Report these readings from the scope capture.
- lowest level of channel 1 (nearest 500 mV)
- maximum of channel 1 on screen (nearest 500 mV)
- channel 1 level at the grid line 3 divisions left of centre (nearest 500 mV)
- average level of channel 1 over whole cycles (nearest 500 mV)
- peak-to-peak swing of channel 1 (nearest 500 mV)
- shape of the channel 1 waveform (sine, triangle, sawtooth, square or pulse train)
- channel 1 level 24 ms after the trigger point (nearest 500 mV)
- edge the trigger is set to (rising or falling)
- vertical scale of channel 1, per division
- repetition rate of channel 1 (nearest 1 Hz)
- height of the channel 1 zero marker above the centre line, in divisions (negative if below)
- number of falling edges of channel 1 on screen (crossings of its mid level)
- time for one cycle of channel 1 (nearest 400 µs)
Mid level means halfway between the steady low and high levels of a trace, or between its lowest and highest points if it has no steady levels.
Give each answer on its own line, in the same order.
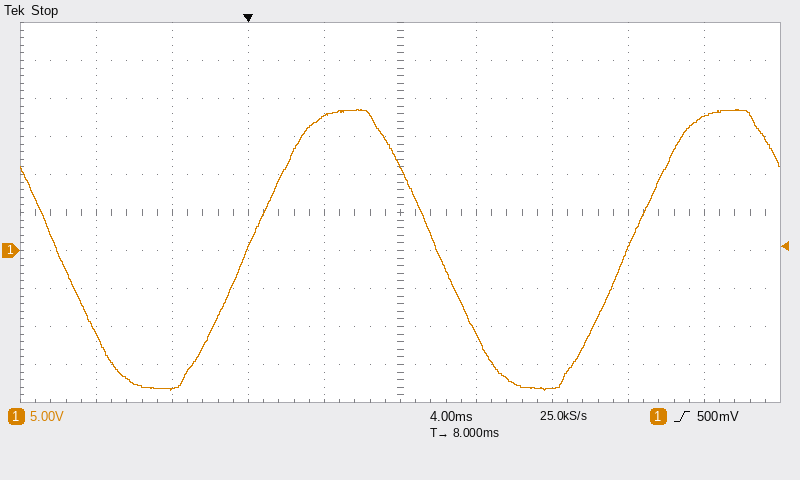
-18.5 V
18.5 V
-18.0 V
0.0 V
37.0 V
sine
17.5 V
rising
5 V
50 Hz
-1.0 div
2
20.0 ms
